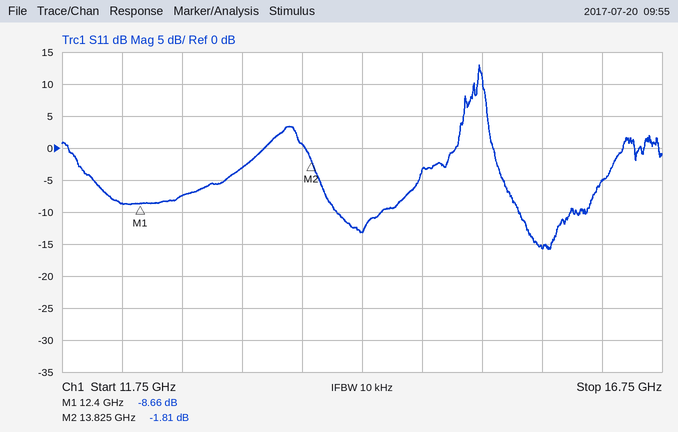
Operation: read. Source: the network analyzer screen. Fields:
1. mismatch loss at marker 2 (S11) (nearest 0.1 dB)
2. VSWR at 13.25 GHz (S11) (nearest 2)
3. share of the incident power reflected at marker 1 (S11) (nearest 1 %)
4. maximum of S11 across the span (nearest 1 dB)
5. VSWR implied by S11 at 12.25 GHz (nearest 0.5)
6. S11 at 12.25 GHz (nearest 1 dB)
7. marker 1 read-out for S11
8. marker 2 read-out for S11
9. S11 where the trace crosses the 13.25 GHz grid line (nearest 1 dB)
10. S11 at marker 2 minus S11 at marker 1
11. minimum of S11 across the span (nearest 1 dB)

4.7 dB
6
14 %
13 dB
2.0
-9 dB
-8.66 dB
-1.81 dB
-3 dB
6.85 dB
-16 dB
